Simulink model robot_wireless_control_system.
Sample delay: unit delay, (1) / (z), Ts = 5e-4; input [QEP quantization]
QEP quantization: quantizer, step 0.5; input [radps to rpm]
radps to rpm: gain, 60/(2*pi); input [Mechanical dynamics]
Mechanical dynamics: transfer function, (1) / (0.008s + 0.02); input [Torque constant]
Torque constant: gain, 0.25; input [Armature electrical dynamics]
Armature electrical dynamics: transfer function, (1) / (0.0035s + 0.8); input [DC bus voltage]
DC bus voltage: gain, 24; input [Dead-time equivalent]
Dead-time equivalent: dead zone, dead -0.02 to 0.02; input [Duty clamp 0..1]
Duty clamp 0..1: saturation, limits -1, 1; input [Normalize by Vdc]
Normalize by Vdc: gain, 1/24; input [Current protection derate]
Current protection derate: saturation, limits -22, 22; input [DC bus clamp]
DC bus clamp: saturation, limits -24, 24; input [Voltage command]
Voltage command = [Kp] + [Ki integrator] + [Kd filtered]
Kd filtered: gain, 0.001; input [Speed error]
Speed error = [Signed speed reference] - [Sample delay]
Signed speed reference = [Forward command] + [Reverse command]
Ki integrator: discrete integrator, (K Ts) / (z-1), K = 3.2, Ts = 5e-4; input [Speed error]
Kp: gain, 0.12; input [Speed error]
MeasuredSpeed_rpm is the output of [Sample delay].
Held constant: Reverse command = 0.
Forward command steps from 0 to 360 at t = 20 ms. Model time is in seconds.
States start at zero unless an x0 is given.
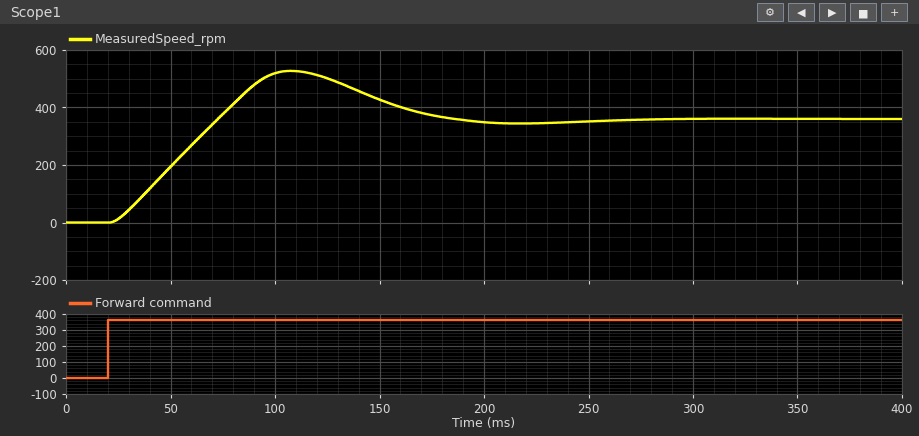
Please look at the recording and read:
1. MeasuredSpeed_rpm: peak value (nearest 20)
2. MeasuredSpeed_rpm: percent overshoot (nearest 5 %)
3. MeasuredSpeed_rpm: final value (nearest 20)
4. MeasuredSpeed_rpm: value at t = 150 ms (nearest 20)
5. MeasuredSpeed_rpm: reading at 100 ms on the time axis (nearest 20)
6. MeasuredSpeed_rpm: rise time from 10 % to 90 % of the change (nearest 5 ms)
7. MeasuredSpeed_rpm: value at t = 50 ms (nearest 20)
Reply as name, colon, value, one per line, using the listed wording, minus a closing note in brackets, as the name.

MeasuredSpeed_rpm: peak value: 520
MeasuredSpeed_rpm: percent overshoot: 45 %
MeasuredSpeed_rpm: final value: 360
MeasuredSpeed_rpm: value at t = 150 ms: 420
MeasuredSpeed_rpm: reading at 100 ms on the time axis: 520
MeasuredSpeed_rpm: rise time from 10 % to 90 % of the change: 40 ms
MeasuredSpeed_rpm: value at t = 50 ms: 200
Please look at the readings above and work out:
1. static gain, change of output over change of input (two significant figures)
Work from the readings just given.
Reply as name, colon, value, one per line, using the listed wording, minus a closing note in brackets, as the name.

static gain, change of output over change of input: 1.0
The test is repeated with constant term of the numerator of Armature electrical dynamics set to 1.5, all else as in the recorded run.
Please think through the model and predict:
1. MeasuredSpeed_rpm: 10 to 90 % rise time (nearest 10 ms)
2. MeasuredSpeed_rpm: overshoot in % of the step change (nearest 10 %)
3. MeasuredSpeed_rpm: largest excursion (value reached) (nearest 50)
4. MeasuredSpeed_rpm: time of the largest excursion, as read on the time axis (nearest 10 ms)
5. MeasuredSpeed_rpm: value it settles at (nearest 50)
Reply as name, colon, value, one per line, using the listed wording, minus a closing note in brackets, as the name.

MeasuredSpeed_rpm: 10 to 90 % rise time: 30 ms
MeasuredSpeed_rpm: overshoot in % of the step change: 40 %
MeasuredSpeed_rpm: largest excursion (value reached): 500
MeasuredSpeed_rpm: time of the largest excursion, as read on the time axis: 80 ms
MeasuredSpeed_rpm: value it settles at: 350
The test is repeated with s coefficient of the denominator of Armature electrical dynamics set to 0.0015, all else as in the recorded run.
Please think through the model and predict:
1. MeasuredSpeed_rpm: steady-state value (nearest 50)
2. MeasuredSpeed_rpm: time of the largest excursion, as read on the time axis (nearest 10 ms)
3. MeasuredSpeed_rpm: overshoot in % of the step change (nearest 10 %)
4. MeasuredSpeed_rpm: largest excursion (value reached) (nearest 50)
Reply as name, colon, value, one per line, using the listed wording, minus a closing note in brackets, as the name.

MeasuredSpeed_rpm: steady-state value: 350
MeasuredSpeed_rpm: time of the largest excursion, as read on the time axis: 100 ms
MeasuredSpeed_rpm: overshoot in % of the step change: 40 %
MeasuredSpeed_rpm: largest excursion (value reached): 500
